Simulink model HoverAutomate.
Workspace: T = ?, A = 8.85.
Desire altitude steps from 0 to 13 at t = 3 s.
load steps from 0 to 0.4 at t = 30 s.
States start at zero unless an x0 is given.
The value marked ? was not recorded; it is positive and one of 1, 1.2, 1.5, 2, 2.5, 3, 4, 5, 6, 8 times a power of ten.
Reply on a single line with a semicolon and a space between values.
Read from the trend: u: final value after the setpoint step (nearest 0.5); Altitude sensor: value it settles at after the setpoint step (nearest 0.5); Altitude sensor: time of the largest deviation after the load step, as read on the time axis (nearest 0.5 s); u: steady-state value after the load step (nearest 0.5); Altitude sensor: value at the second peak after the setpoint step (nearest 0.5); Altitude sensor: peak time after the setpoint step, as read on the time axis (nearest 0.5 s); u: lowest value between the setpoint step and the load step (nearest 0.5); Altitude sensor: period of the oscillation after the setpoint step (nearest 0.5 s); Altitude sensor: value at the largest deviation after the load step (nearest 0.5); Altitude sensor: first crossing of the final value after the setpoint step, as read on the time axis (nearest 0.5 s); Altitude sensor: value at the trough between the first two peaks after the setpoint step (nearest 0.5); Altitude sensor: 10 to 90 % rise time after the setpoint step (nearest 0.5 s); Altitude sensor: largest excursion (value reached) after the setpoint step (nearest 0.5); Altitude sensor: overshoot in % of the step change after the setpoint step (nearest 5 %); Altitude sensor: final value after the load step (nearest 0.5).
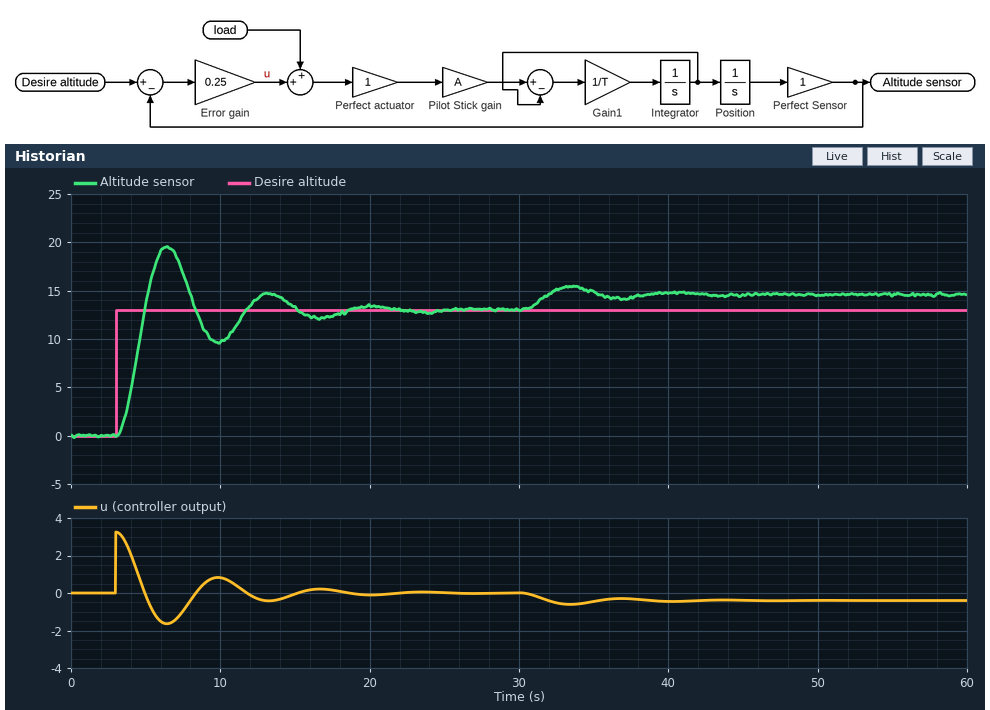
0.0; 13.0; 33.5 s; -0.5; 14.5; 6.5 s; -1.5; 7.0 s; 15.5; 5.0 s; 9.5; 1.5 s; 19.5; 50 %; 14.5
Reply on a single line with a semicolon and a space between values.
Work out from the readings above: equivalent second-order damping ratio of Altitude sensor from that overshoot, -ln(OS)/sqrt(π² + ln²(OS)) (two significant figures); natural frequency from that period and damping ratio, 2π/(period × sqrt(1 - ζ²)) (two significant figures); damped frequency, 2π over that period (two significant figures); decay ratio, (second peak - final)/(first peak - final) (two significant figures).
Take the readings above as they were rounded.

0.22; 0.92 rad/s; 0.90 rad/s; 0.23
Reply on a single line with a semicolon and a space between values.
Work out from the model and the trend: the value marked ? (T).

2.5
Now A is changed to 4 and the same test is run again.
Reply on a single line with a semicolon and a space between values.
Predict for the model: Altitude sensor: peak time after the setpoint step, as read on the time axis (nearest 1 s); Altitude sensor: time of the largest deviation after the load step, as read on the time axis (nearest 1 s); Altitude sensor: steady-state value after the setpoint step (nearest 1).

8 s; 35 s; 13
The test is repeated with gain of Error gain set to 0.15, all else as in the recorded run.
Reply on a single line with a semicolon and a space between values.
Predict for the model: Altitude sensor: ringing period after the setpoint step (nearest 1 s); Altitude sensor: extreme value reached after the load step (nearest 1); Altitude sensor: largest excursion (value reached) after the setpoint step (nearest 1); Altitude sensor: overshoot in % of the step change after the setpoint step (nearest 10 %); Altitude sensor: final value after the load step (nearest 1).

9 s; 17; 18; 40 %; 16
